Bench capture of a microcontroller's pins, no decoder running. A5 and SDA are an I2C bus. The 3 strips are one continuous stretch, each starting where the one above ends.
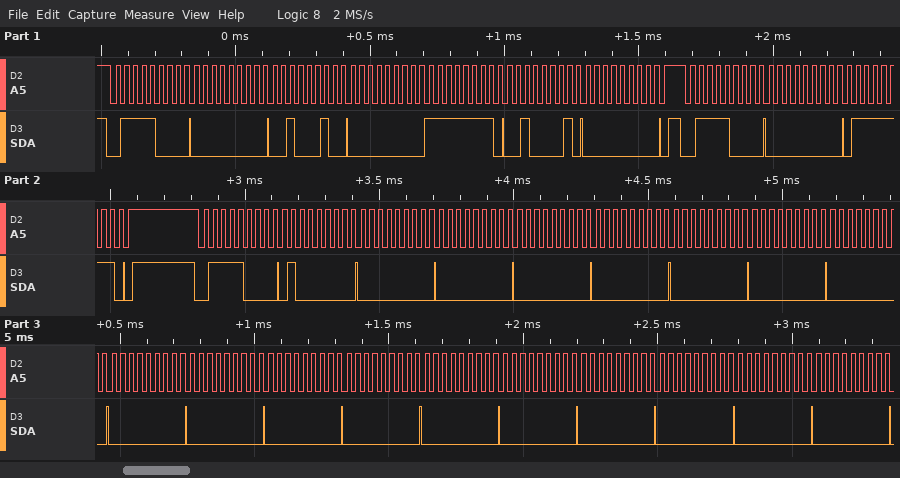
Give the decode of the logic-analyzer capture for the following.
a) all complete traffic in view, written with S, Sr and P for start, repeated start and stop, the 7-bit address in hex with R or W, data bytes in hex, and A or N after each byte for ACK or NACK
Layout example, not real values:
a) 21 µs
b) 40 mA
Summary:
a) S 3CW A 00 A 22 A 00 A FF A 21 A 00 A P S 3CW A 00 A 7F A P S 3CW A 40 A 00 A 00 A 00 A 00 A 00 A 00 A 00 A 00 A 00 A 00 A 00 A 00 A 00 A 00 A 00 A 00 A 00 A
